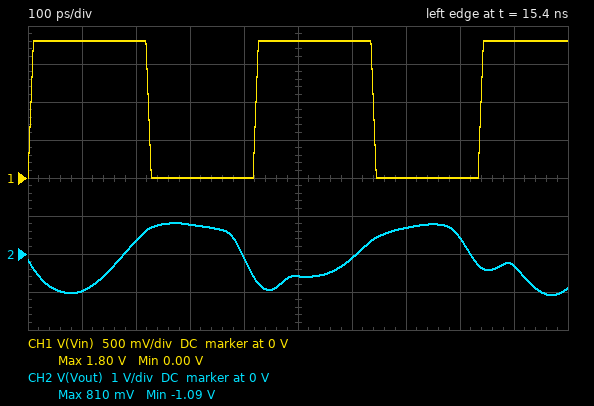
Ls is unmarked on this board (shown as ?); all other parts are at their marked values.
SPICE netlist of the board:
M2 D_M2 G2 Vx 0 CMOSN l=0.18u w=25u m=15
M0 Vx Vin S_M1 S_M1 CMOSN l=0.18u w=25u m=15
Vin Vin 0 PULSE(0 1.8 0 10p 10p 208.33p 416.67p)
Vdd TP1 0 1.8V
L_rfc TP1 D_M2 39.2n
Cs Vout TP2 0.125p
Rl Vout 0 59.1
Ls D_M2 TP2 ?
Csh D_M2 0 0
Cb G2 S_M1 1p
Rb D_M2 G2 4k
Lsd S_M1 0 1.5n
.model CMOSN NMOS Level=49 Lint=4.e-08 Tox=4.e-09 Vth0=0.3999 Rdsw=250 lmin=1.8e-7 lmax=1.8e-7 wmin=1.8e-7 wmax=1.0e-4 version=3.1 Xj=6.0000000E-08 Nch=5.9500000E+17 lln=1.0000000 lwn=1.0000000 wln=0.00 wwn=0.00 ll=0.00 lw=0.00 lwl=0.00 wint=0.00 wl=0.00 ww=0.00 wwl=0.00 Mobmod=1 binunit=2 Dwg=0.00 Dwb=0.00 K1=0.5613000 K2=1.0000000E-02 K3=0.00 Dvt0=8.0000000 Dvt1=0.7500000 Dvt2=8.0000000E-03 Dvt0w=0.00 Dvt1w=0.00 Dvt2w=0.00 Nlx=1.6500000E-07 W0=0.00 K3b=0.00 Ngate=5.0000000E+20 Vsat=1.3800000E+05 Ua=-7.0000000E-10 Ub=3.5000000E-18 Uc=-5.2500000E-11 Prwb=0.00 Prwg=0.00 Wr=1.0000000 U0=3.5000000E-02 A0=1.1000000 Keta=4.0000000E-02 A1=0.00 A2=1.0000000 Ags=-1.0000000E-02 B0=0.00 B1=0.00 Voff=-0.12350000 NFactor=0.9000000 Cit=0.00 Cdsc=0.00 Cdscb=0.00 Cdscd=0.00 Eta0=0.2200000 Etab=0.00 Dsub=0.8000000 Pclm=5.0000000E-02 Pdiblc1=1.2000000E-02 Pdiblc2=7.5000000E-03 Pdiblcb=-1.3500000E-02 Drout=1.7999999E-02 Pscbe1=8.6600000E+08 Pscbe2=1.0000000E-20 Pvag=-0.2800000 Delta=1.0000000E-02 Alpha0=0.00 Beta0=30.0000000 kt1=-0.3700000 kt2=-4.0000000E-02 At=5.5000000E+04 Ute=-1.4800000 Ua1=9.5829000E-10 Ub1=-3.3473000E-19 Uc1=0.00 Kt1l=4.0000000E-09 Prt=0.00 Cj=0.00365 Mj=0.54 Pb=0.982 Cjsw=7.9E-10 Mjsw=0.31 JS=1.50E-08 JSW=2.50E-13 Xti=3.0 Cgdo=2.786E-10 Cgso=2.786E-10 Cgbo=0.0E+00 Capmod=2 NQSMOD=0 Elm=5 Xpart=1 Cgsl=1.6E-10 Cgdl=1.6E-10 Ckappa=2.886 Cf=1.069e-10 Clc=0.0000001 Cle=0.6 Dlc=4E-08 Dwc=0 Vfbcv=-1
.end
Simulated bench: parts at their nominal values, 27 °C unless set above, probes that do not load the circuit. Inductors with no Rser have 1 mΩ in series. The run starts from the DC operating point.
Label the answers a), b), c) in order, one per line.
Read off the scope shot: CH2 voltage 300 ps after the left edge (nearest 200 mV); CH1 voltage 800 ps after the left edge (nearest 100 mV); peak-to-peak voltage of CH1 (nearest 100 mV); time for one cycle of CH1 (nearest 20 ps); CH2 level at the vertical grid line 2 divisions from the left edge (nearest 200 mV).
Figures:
a) 800 mV
b) 0 V
c) 1.8 V
d) 420 ps
e) 400 mV
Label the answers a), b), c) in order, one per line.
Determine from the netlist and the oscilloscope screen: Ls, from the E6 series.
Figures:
a) 22 nH
